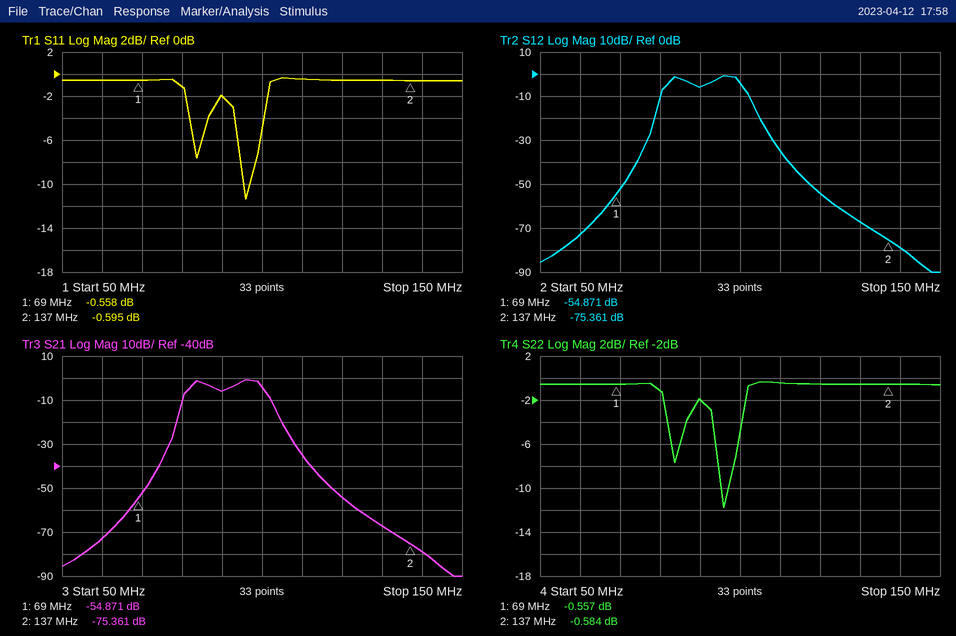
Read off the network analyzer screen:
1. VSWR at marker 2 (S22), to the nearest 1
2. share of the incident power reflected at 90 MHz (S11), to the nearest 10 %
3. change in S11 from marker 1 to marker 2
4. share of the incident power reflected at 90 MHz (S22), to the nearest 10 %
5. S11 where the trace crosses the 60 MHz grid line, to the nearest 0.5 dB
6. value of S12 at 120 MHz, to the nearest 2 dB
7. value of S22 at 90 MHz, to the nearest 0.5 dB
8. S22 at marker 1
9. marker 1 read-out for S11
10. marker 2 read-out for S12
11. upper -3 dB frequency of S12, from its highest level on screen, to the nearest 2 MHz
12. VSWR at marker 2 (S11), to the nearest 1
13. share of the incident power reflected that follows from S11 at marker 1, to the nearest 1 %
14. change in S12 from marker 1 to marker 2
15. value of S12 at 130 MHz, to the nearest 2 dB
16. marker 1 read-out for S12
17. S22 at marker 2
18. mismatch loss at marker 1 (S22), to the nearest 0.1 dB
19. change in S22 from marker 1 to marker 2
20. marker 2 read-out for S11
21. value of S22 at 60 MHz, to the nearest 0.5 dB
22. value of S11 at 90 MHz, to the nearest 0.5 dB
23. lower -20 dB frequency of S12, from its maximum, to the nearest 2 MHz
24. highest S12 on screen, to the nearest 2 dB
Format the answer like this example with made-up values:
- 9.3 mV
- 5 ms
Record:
- 30
- 60 %
- -0.037 dB
- 60 %
- -0.5 dB
- -54 dB
- -2.0 dB
- -0.557 dB
- -0.558 dB
- -75.361 dB
- 100 MHz
- 29
- 88 %
- -20.490 dB
- -68 dB
- -54.871 dB
- -0.584 dB
- 9.2 dB
- -0.027 dB
- -0.595 dB
- -0.5 dB
- -2.0 dB
- 78 MHz
- 0 dB
